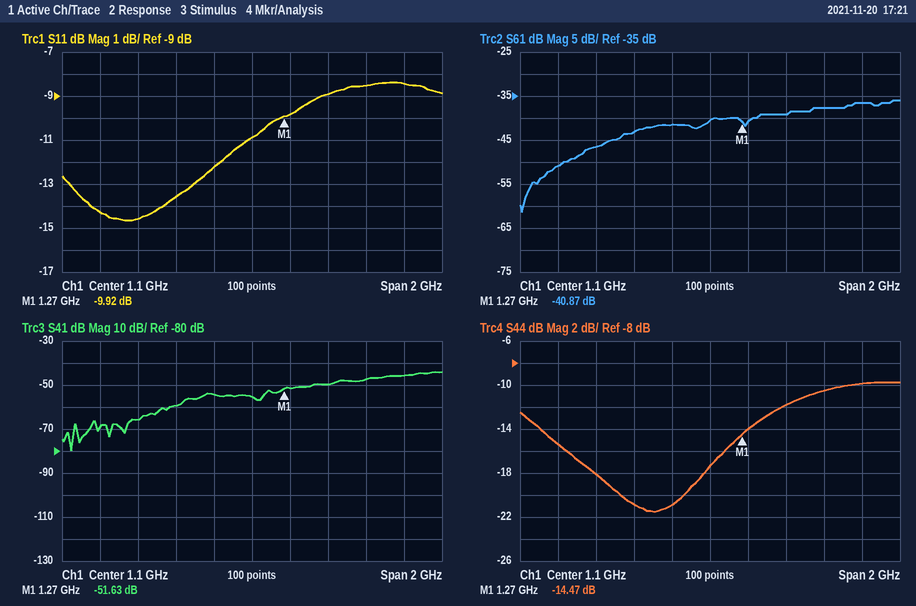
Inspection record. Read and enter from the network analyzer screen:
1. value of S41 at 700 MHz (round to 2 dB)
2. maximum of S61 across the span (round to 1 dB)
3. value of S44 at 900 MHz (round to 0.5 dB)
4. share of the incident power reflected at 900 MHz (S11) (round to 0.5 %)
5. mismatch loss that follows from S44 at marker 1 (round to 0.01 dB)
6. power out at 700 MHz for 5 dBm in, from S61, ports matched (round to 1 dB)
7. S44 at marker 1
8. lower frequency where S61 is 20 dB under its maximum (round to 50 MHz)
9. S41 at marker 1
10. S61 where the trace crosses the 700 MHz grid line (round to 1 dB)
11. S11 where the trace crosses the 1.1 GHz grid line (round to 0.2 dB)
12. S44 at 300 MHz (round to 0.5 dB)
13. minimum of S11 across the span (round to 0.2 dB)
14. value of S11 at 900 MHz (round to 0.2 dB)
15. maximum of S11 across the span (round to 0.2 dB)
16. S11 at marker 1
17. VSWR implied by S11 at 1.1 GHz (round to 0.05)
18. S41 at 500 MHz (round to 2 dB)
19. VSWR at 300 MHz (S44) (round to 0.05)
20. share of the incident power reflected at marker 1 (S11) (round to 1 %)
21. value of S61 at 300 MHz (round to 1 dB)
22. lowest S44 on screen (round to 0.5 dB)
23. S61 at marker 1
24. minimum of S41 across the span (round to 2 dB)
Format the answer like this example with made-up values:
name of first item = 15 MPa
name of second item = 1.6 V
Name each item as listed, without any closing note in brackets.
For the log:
value of S41 at 700 MHz = -60 dB
maximum of S61 across the span = -36 dB
value of S44 at 900 MHz = -21.0 dB
share of the incident power reflected at 900 MHz (S11) = 6.0 %
mismatch loss that follows from S44 at marker 1 = 0.16 dB
power out at 700 MHz for 5 dBm in, from S61, ports matched = -38 dBm
S44 at marker 1 = -14.47 dB
lower frequency where S61 is 20 dB under its maximum = 150 MHz
S41 at marker 1 = -51.63 dB
S61 where the trace crosses the 700 MHz grid line = -43 dB
S11 where the trace crosses the 1.1 GHz grid line = -10.8 dB
S44 at 300 MHz = -15.5 dB
minimum of S11 across the span = -14.6 dB
value of S11 at 900 MHz = -12.2 dB
maximum of S11 across the span = -8.4 dB
S11 at marker 1 = -9.92 dB
VSWR implied by S11 at 1.1 GHz = 1.80
S41 at 500 MHz = -66 dB
VSWR at 300 MHz (S44) = 1.40
share of the incident power reflected at marker 1 (S11) = 10 %
value of S61 at 300 MHz = -51 dB
lowest S44 on screen = -21.5 dB
S61 at marker 1 = -40.87 dB
minimum of S41 across the span = -80 dB
